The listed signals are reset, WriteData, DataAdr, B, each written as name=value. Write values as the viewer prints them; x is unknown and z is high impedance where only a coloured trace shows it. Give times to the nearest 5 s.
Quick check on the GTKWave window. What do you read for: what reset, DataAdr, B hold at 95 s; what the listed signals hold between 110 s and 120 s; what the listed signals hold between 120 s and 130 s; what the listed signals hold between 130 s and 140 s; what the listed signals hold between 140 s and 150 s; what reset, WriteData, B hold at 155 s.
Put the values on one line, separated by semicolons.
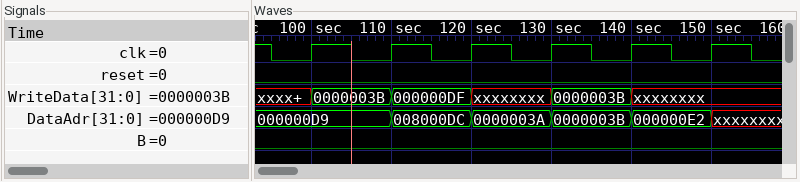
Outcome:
reset=0, DataAdr=000000D9, B=0; reset=0, WriteData=000000DF, DataAdr=008000DC, B=0; reset=0, WriteData=xxxxxxxx, DataAdr=0000003A, B=0; reset=0, WriteData=0000003B, DataAdr=0000003B, B=0; reset=0, WriteData=xxxxxxxx, DataAdr=000000E2, B=0; reset=0, WriteData=xxxxxxxx, B=0
